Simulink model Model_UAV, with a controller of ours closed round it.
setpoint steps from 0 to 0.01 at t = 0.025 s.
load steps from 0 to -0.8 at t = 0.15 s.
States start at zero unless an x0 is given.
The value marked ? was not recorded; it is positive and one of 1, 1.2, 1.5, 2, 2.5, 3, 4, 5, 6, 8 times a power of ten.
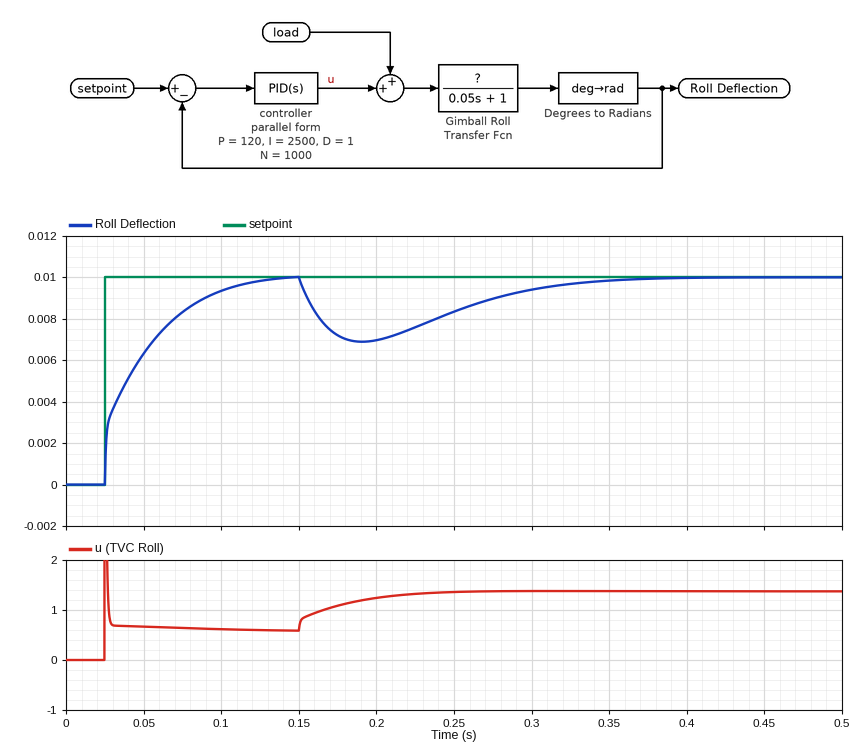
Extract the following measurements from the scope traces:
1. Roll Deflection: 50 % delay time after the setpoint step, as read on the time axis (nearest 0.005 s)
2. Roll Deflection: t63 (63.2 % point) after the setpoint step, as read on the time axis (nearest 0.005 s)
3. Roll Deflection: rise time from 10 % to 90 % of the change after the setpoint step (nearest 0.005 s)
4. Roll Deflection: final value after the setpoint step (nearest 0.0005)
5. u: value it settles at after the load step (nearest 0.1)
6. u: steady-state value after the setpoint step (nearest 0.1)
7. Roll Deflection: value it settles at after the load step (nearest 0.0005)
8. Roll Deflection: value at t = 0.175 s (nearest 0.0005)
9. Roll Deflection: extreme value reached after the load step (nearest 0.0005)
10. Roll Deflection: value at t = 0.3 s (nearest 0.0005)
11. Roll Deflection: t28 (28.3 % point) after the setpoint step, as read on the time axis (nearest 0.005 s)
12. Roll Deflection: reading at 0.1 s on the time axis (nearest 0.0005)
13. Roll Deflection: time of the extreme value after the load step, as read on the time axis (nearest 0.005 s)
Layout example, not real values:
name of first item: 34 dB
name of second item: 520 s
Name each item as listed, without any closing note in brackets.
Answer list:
Roll Deflection: 50 % delay time after the setpoint step, as read on the time axis: 0.040 s
Roll Deflection: t63 (63.2 % point) after the setpoint step, as read on the time axis: 0.050 s
Roll Deflection: rise time from 10 % to 90 % of the change after the setpoint step: 0.065 s
Roll Deflection: final value after the setpoint step: 0.0100
u: value it settles at after the load step: 1.4
u: steady-state value after the setpoint step: 0.6
Roll Deflection: value it settles at after the load step: 0.0100
Roll Deflection: value at t = 0.175 s: 0.0070
Roll Deflection: extreme value reached after the load step: 0.0070
Roll Deflection: value at t = 0.3 s: 0.0095
Roll Deflection: t28 (28.3 % point) after the setpoint step, as read on the time axis: 0.025 s
Roll Deflection: reading at 0.1 s on the time axis: 0.0095
Roll Deflection: time of the extreme value after the load step, as read on the time axis: 0.190 s
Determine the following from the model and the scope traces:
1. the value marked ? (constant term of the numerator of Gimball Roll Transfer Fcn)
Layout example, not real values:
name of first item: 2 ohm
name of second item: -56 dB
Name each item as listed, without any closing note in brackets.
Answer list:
the value marked ?: 1
